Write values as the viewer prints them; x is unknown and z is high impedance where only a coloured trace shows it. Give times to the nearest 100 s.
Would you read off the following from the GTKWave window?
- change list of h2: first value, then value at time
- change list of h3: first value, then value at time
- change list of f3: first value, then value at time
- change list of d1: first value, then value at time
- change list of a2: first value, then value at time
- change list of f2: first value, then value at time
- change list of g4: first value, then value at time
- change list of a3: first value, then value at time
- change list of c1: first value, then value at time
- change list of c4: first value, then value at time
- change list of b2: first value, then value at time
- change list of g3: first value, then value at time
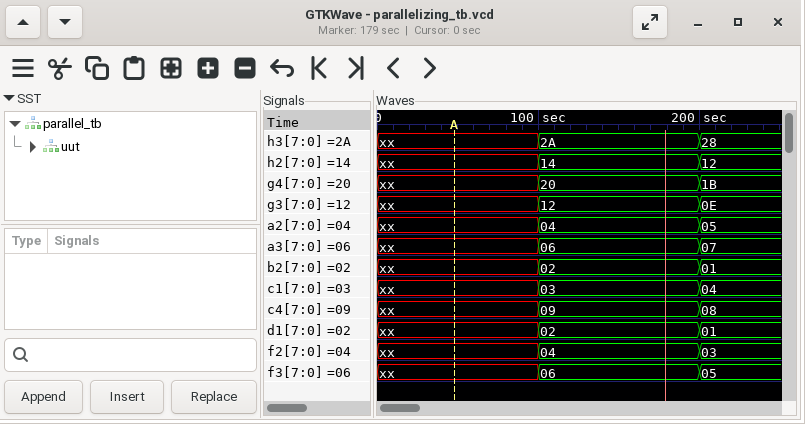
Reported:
xx, 14 at 100 s, 12 at 200 s
xx, 2A at 100 s, 28 at 200 s
xx, 06 at 100 s, 05 at 200 s
xx, 02 at 100 s, 01 at 200 s
xx, 04 at 100 s, 05 at 200 s
xx, 04 at 100 s, 03 at 200 s
xx, 20 at 100 s, 1B at 200 s
xx, 06 at 100 s, 07 at 200 s
xx, 03 at 100 s, 04 at 200 s
xx, 09 at 100 s, 08 at 200 s
xx, 02 at 100 s, 01 at 200 s
xx, 12 at 100 s, 0E at 200 s
